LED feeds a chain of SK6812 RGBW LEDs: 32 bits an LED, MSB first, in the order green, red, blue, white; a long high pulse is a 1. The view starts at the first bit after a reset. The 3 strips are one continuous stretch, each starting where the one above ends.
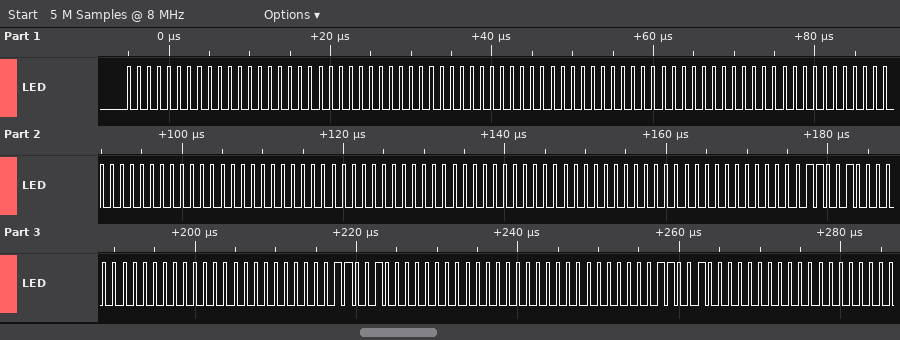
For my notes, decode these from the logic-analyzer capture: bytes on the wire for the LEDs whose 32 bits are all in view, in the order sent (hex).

00 00 00 00 00 00 00 00 00 00 00 00 00 00 00 00 00 00 32 00 00 00 32 00 00 00 32 00
